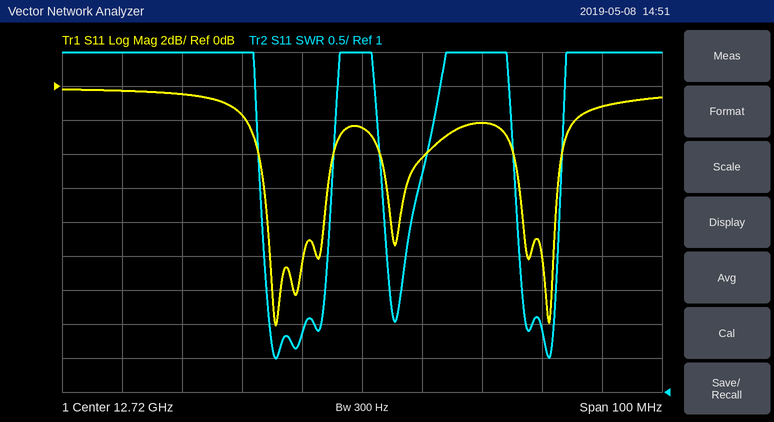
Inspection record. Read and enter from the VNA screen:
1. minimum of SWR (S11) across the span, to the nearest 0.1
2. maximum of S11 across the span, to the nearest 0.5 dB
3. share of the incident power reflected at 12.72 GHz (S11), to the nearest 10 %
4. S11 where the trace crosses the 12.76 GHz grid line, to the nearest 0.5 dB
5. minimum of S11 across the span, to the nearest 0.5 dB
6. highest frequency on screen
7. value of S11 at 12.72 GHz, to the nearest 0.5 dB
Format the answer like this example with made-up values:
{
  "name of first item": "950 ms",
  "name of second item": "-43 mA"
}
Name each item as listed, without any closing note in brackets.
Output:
{
  "minimum of SWR (S11) across the span, to the nearest 0.1": "1.5",
  "maximum of S11 across the span, to the nearest 0.5 dB": "0.0 dB",
  "share of the incident power reflected at 12.72 GHz (S11), to the nearest 10 %": "60 %",
  "S11 where the trace crosses the 12.76 GHz grid line, to the nearest 0.5 dB": "-1.0 dB",
  "minimum of S11 across the span, to the nearest 0.5 dB": "-14.0 dB",
  "highest frequency on screen": "12.77 GHz",
  "value of S11 at 12.72 GHz, to the nearest 0.5 dB": "-2.5 dB"
}
